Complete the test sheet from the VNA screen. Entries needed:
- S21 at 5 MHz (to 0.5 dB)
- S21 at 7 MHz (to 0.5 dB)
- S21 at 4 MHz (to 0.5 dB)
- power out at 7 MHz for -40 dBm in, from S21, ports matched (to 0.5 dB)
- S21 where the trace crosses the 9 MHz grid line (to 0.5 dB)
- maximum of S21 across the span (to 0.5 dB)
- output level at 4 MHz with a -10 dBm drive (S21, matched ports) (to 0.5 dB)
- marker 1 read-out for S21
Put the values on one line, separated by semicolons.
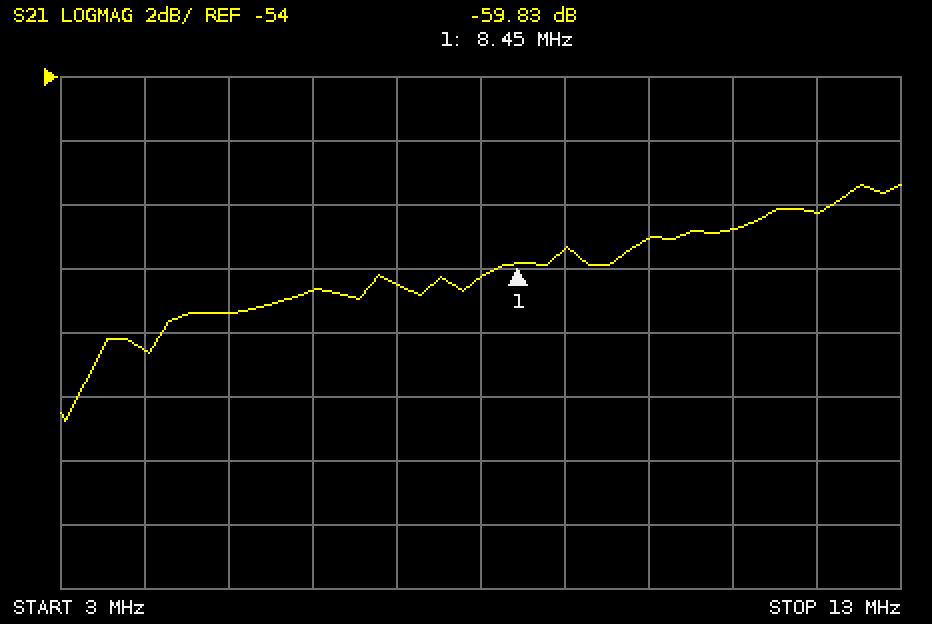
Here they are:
-61.5 dB; -60.5 dB; -62.5 dB; -100.5 dBm; -59.5 dB; -57.5 dB; -72.5 dBm; -59.83 dB
